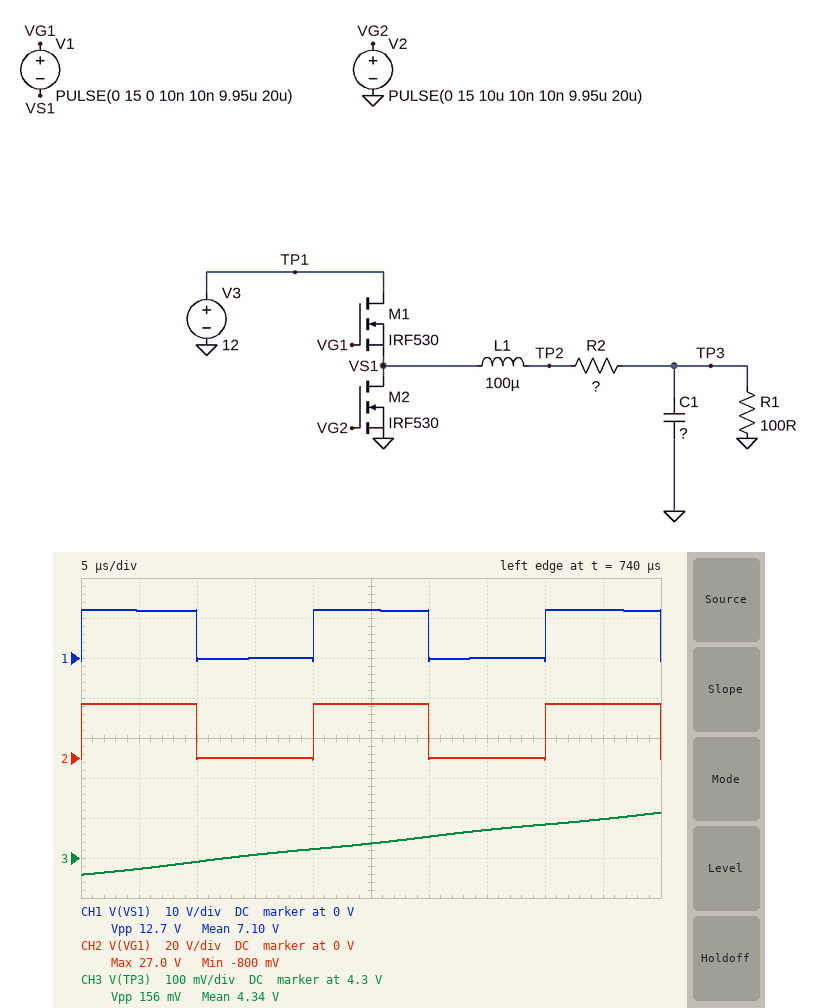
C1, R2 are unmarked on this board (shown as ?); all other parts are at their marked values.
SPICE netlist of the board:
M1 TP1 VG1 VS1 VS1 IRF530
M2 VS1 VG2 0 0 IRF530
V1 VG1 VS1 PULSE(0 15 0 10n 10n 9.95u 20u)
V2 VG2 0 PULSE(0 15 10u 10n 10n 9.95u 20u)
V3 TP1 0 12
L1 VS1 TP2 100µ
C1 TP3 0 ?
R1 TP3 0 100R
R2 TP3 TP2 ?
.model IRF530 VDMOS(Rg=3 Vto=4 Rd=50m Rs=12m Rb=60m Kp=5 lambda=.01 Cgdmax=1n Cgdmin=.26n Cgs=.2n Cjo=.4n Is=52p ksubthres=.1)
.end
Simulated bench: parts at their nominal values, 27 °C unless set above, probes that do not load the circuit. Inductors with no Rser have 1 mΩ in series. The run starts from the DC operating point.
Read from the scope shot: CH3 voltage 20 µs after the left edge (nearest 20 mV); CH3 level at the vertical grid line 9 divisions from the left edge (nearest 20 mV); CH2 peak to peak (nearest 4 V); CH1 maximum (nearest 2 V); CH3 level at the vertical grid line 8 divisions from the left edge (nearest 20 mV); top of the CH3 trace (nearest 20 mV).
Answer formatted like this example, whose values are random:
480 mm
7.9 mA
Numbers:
4.32 V
4.40 V
28 V
12 V
4.38 V
4.42 V
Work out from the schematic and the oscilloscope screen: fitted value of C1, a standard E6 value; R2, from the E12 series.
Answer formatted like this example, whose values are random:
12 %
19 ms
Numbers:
470 µF
1.2 Ω
